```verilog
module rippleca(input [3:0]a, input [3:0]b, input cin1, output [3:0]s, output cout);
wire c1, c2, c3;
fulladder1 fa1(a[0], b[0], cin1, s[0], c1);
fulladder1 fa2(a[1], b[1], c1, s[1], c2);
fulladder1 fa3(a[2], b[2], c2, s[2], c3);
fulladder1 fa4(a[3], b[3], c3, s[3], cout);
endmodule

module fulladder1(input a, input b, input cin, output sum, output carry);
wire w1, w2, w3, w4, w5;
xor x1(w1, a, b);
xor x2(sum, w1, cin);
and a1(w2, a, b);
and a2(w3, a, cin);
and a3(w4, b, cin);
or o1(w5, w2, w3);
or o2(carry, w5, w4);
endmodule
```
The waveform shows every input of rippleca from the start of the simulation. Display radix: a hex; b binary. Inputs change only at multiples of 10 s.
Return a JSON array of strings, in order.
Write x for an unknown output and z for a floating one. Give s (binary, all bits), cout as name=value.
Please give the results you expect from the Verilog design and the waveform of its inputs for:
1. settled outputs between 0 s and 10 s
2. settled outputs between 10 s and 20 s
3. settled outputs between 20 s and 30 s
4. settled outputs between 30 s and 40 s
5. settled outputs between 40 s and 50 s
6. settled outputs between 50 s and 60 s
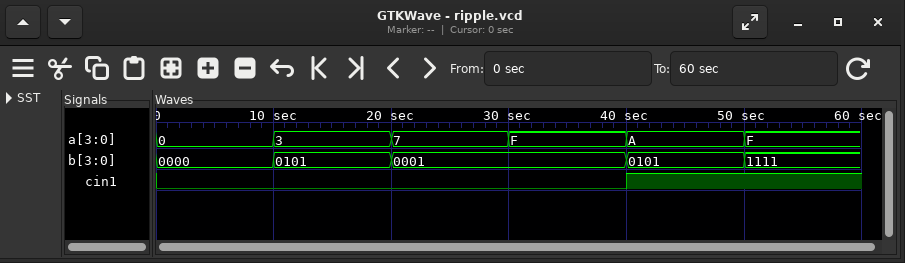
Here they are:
["s=0000, cout=0", "s=1000, cout=0", "s=1000, cout=0", "s=0000, cout=1", "s=0000, cout=1", "s=1111, cout=1"]
